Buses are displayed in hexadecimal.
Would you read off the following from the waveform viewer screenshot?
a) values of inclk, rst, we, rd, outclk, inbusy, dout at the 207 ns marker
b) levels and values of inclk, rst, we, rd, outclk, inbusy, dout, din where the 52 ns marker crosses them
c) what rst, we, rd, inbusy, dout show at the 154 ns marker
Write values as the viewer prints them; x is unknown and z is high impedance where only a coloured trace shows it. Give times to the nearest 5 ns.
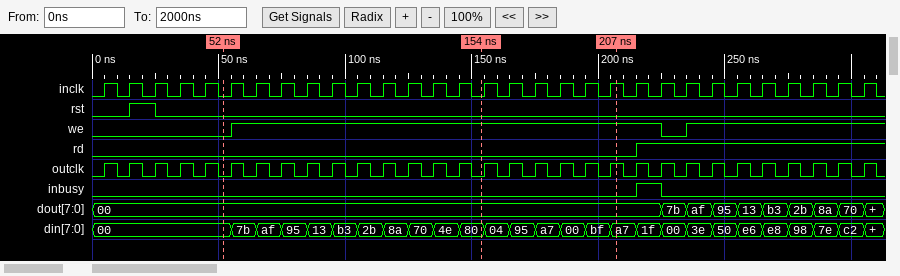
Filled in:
inclk=1, rst=0, we=1, rd=0, outclk=1, inbusy=0, dout=00
inclk=0, rst=0, we=0, rd=0, outclk=0, inbusy=0, dout=00, din=00
rst=0, we=1, rd=0, inbusy=0, dout=00
